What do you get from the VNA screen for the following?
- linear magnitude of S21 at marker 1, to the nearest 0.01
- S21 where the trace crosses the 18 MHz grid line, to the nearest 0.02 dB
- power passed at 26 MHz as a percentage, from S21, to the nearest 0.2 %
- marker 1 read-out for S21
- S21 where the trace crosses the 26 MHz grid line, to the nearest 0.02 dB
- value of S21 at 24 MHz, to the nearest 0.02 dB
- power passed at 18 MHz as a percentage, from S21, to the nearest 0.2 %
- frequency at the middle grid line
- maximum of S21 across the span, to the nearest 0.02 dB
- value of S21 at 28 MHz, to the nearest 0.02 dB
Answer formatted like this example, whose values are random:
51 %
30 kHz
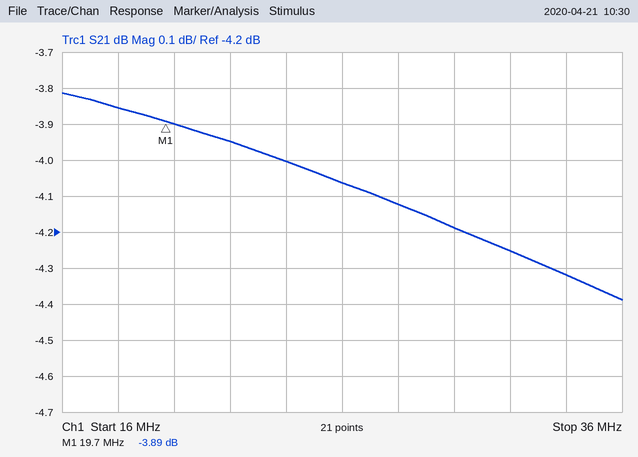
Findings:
0.64
-3.86 dB
39.2 %
-3.89 dB
-4.06 dB
-4.00 dB
41.2 %
26 MHz
-3.82 dB
-4.12 dB
